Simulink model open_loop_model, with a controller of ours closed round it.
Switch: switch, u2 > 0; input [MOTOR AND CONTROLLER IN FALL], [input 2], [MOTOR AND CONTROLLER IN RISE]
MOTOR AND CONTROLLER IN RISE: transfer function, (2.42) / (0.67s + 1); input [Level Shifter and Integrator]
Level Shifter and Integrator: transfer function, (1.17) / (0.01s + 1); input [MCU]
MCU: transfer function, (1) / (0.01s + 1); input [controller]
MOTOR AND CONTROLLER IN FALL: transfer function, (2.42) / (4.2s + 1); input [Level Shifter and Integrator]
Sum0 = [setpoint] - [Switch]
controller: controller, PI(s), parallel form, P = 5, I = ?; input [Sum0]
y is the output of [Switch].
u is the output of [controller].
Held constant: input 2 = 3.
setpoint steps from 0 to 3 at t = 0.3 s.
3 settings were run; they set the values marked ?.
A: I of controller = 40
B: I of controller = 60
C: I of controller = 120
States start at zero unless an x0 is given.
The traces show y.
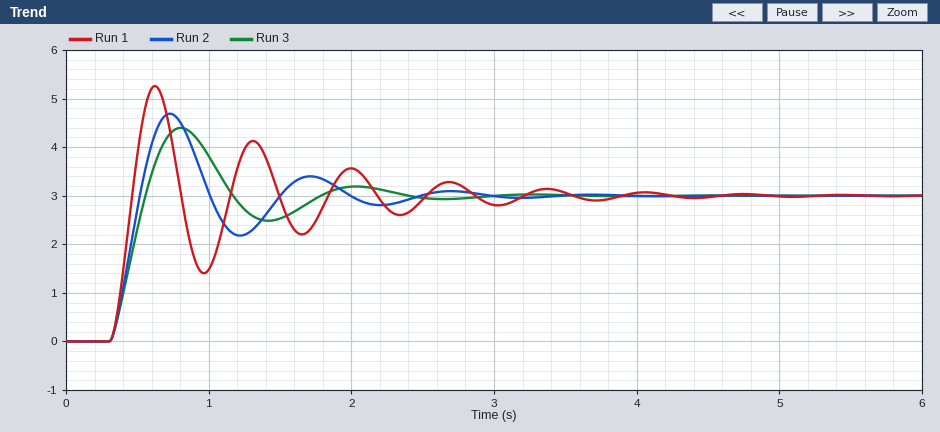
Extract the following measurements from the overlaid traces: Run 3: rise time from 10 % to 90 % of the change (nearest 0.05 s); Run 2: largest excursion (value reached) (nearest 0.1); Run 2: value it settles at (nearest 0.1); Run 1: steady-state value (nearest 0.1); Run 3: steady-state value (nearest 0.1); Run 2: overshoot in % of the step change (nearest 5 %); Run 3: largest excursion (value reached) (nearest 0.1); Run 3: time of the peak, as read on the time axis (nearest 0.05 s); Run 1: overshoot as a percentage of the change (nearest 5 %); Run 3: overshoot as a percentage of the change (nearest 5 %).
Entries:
0.20 s
4.7
3.0
3.0
3.0
55 %
4.4
0.80 s
75 %
45 %
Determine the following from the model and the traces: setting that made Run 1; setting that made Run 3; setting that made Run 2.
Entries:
C
A
B
